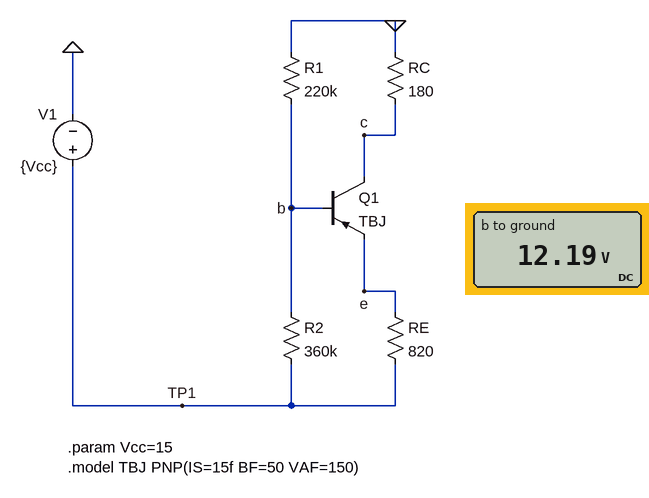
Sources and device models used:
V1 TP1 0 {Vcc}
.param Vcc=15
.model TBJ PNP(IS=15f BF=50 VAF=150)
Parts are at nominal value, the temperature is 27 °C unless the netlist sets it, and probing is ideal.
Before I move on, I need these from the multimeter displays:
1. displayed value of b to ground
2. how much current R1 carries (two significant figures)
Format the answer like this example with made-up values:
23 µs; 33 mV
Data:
12.19 V; 55 µA
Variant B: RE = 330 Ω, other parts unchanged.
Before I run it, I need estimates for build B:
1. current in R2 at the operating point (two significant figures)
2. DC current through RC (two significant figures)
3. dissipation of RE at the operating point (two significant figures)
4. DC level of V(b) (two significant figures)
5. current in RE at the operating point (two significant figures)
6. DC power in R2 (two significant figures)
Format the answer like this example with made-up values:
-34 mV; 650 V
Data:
4.7 µA; 3.0 mA; 3.1 mW; 13 V; 3.1 mA; 7.9 µW
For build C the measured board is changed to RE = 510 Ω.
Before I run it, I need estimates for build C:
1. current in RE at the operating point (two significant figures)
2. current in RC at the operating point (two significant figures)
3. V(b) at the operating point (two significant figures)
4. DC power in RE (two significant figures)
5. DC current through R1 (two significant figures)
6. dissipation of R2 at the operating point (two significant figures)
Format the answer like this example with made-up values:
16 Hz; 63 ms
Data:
2.9 mA; 2.8 mA; 13 V; 4.3 mW; 58 µA; 13 µW
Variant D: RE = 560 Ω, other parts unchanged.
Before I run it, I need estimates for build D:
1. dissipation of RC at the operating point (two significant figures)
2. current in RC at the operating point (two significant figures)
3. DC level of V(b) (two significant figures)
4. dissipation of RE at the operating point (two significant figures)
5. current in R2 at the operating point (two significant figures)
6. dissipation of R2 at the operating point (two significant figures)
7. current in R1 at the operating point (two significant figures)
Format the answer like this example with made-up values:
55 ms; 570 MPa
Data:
1.4 mW; 2.8 mA; 13 V; 4.5 mW; 6.3 µA; 14 µW; 58 µA
